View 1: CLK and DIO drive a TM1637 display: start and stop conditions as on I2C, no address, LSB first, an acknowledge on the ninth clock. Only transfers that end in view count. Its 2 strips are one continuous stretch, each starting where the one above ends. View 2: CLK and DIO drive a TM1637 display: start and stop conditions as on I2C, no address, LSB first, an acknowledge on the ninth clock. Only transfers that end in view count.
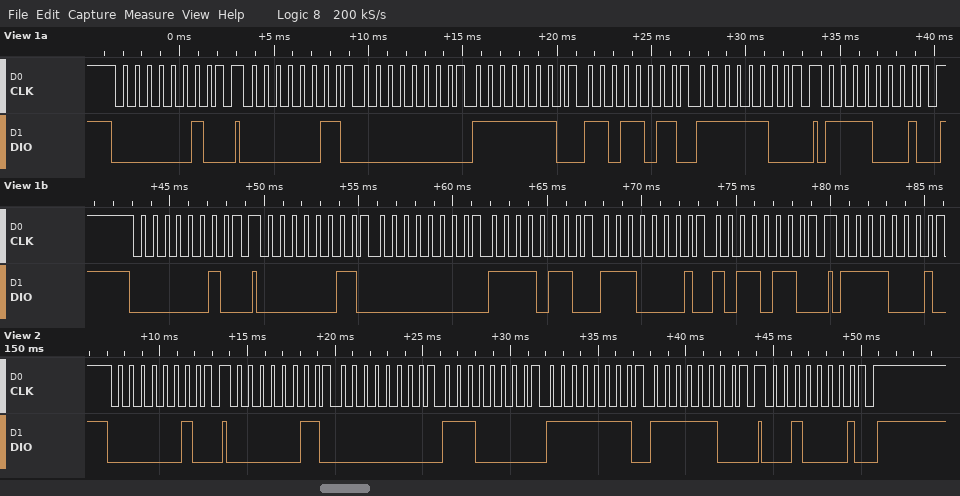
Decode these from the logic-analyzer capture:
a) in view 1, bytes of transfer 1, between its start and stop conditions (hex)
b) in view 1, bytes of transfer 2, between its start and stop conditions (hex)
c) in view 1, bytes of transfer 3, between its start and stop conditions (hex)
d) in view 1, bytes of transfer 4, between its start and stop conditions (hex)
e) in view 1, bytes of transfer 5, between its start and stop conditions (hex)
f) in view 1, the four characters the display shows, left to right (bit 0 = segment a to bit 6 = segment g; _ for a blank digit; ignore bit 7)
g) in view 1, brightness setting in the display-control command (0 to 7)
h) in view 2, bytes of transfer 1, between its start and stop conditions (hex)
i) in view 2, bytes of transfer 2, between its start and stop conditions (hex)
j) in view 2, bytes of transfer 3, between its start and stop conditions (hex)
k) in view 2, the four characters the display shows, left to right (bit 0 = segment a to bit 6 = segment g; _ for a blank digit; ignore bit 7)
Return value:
40
C0 00 7F DB 3F
8F
40
C0 00 6F 87 6D
_975
7
40
C0 00 07 FF 3F
84
_780
